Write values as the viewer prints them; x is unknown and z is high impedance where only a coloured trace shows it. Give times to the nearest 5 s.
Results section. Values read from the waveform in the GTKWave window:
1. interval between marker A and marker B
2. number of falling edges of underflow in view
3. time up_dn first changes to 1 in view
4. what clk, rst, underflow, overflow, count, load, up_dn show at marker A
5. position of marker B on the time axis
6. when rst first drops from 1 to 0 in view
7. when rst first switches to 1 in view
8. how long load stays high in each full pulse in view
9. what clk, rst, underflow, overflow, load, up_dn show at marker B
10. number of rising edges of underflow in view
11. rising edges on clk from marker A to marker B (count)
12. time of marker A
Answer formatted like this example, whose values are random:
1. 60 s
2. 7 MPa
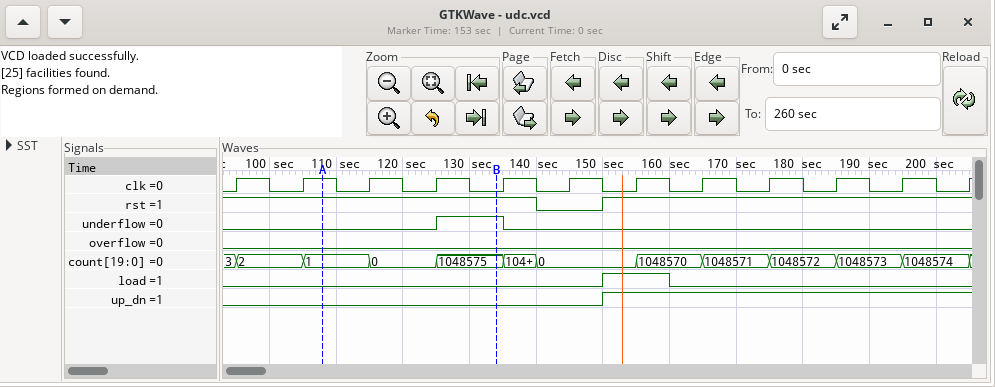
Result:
1. 25 s
2. 1
3. 150 s
4. clk=1, rst=1, underflow=0, overflow=0, count=1, load=0, up_dn=0
5. 135 s
6. 140 s
7. 150 s
8. 10 s
9. clk=0, rst=1, underflow=1, overflow=0, load=0, up_dn=0
10. 1
11. 2
12. 110 s
